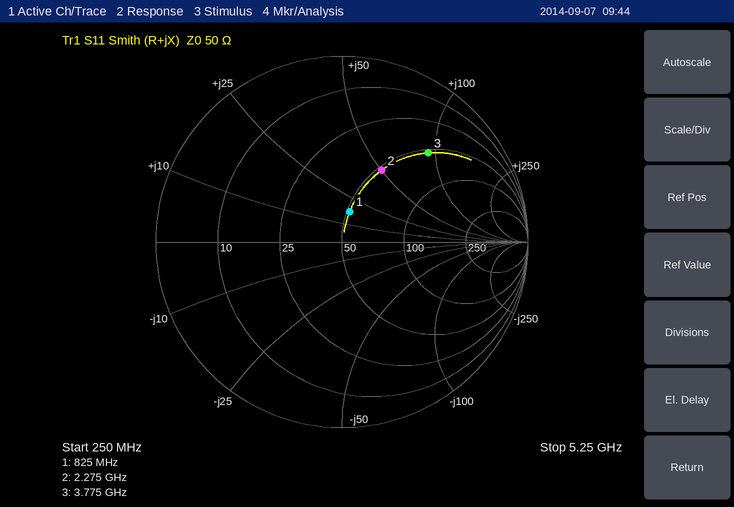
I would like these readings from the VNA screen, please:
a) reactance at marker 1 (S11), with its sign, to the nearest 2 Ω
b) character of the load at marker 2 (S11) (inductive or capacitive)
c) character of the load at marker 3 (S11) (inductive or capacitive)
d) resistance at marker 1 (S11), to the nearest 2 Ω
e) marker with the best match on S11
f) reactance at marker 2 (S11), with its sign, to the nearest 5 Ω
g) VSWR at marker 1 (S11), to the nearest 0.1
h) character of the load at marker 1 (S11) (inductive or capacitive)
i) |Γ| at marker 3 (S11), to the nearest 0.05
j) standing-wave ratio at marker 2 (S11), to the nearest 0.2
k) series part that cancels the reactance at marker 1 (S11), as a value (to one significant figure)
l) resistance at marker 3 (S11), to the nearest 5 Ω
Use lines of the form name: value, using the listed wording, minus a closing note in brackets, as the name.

reactance at marker 1 (S11), with its sign, to the nearest 2 Ω: +18 Ω
character of the load at marker 2 (S11): inductive
character of the load at marker 3 (S11): inductive
resistance at marker 1 (S11), to the nearest 2 Ω: 52 Ω
marker with the best match on S11: marker 1
reactance at marker 2 (S11), with its sign, to the nearest 5 Ω: +50 Ω
VSWR at marker 1 (S11), to the nearest 0.1: 1.4
character of the load at marker 1 (S11): inductive
|Γ| at marker 3 (S11), to the nearest 0.05: 0.65
standing-wave ratio at marker 2 (S11), to the nearest 0.2: 2.6
series part that cancels the reactance at marker 1 (S11), as a value: 10 pF
resistance at marker 3 (S11), to the nearest 5 Ω: 55 Ω
